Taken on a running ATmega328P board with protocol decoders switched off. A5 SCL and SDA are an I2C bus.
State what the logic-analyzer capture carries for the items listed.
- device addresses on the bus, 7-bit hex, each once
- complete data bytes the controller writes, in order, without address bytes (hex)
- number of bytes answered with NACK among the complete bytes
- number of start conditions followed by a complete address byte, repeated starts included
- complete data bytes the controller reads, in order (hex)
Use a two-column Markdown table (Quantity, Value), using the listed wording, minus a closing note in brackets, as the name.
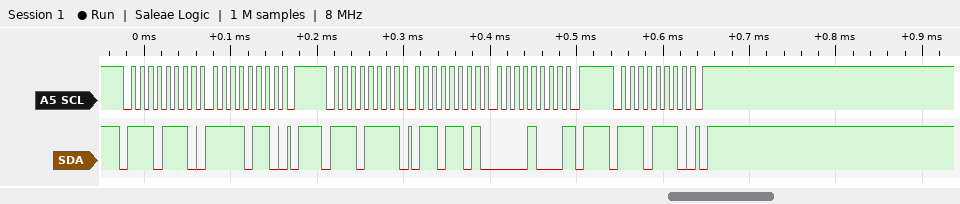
| Quantity | Value |
|---|---|
| device addresses on the bus, 7-bit hex, each once | 0x77 |
| complete data bytes the controller writes, in order, without address bytes | F6 |
| number of bytes answered with NACK among the complete bytes | 1 |
| number of start conditions followed by a complete address byte, repeated starts included | 3 |
| complete data bytes the controller reads, in order | 6D 08 |
